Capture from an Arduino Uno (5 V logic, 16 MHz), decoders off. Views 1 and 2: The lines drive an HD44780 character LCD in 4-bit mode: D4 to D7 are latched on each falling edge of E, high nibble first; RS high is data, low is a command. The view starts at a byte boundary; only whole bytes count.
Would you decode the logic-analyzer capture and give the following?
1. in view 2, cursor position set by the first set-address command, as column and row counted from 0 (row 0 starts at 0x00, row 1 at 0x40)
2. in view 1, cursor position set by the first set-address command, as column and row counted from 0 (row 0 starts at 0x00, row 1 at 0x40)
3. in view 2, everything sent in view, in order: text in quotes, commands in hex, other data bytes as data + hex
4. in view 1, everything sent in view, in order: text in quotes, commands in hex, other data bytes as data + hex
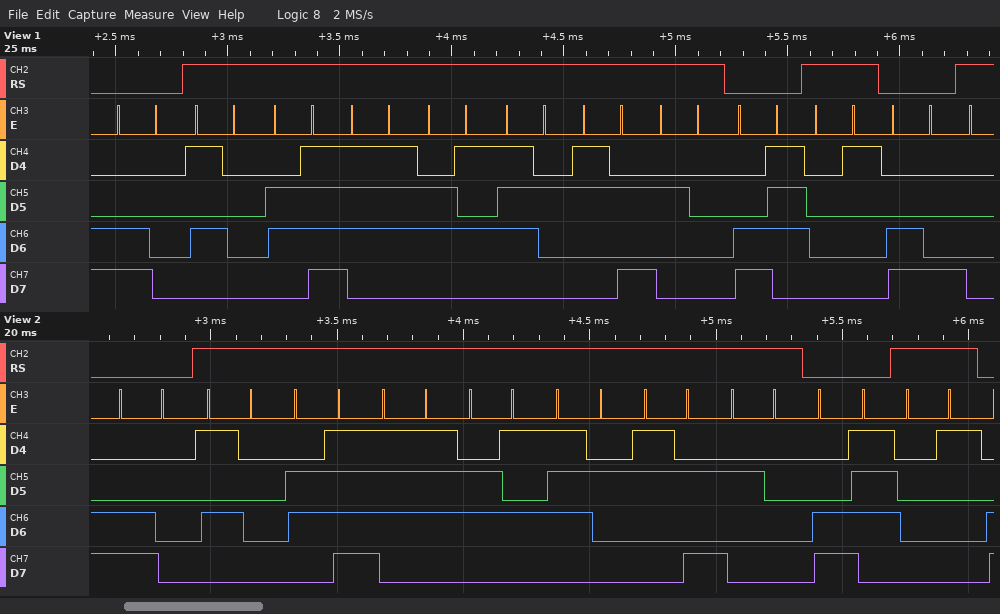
column 0, row 1
column 0, row 1
0xC0 "Power: " 0xC7 data 01
0xC0 "Power: " 0xC7 data 01 0xC8
